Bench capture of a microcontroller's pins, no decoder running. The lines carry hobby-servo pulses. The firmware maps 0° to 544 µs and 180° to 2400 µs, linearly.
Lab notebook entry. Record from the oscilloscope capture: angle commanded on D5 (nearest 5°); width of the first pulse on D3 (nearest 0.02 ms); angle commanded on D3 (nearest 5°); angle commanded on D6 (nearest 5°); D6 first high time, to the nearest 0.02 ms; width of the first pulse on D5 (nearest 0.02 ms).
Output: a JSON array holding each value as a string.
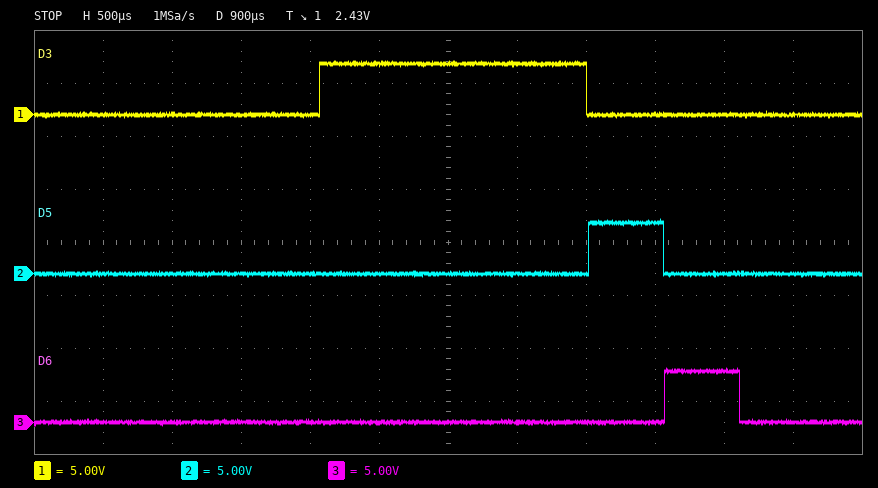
["0°", "1.94 ms", "135°", "0°", "0.54 ms", "0.54 ms"]
